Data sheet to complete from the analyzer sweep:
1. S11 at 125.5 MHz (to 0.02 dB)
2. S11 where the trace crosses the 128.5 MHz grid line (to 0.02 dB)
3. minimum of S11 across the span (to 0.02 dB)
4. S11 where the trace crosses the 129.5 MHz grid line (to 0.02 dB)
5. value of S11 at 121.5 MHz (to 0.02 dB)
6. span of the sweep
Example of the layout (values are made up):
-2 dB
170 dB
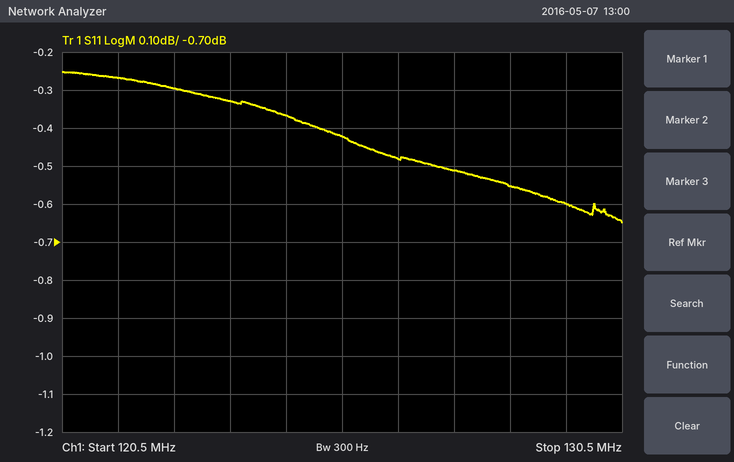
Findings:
-0.42 dB
-0.56 dB
-0.64 dB
-0.60 dB
-0.26 dB
10 MHz
